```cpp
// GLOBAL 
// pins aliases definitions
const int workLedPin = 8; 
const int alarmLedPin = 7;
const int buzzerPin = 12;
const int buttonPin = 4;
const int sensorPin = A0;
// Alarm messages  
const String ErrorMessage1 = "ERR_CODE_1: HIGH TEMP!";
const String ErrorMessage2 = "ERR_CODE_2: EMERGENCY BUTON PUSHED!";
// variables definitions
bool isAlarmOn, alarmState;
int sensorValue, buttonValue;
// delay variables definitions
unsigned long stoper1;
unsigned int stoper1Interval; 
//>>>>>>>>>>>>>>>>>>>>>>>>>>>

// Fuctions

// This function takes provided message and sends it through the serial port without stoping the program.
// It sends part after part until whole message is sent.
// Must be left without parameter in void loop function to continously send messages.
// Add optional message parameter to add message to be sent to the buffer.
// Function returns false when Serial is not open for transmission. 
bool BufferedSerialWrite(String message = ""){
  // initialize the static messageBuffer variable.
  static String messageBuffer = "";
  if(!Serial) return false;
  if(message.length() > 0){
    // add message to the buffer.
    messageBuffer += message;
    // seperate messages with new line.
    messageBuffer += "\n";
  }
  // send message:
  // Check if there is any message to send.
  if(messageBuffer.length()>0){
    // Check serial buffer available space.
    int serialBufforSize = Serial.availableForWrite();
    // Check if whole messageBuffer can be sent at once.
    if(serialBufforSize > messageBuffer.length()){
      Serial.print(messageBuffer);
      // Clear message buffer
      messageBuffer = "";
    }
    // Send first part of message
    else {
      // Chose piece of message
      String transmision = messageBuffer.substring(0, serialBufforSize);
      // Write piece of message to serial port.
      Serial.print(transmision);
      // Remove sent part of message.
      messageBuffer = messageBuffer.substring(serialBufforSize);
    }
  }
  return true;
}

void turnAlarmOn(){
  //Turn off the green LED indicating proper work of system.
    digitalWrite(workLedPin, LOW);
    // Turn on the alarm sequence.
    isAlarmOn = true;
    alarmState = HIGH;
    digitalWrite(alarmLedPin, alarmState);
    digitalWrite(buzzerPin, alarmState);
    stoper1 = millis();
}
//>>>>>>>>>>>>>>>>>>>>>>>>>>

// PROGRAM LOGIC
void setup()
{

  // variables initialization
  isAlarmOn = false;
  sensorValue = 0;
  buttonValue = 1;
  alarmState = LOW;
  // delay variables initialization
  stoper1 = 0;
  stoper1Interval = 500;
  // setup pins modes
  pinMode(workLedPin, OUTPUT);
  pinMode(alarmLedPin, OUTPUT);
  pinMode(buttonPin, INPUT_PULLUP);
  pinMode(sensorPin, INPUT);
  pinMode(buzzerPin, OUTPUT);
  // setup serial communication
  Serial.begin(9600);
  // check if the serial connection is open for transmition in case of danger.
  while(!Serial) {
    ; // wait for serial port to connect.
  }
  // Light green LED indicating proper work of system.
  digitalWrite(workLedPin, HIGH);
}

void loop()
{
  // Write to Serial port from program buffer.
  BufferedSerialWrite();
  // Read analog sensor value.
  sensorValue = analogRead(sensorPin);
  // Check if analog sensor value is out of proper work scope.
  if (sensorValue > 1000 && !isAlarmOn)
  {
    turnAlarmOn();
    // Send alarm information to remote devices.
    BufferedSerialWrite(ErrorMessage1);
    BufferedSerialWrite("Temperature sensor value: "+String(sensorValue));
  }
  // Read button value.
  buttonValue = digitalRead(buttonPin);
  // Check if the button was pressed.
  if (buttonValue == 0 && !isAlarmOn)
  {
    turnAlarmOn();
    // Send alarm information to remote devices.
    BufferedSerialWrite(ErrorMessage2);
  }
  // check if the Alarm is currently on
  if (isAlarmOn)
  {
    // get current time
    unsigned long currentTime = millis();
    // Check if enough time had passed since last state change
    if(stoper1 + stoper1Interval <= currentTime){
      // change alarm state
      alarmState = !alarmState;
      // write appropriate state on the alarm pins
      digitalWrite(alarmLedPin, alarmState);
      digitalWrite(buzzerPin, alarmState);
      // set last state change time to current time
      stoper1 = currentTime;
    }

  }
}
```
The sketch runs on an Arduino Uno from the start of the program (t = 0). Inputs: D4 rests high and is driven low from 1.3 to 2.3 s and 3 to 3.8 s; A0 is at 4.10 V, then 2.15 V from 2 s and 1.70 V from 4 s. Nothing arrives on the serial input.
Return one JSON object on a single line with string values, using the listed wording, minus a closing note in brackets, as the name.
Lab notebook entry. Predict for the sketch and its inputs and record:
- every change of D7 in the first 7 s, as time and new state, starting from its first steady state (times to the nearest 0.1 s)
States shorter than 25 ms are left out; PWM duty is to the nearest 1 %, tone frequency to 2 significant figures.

{"every change of D7 in the first 7 s, as time and new state, starting from its first steady state": "0 s low; 1.3 s high; 1.8 s low; 2.3 s high; 2.8 s low; 3.3 s high; 3.8 s low; 4.3 s high; 4.8 s low; 5.3 s high; 5.8 s low; 6.3 s high; 6.8 s low"}
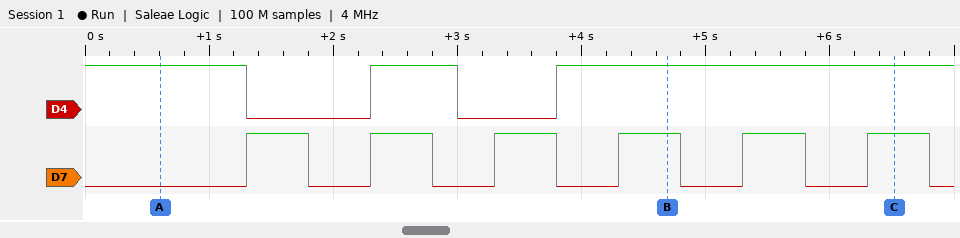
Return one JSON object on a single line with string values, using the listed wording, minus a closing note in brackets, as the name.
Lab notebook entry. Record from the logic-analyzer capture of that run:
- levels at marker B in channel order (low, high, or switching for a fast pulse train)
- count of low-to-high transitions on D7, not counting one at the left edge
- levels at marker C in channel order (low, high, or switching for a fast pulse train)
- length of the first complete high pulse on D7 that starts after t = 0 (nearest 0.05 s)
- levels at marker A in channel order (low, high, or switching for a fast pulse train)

{"levels at marker B in channel order": "D4 high, D7 high", "count of low-to-high transitions on D7, not counting one at the left edge": "6", "levels at marker C in channel order": "D4 high, D7 high", "length of the first complete high pulse on D7 that starts after t = 0": "0.50 s", "levels at marker A in channel order": "D4 high, D7 low"}
